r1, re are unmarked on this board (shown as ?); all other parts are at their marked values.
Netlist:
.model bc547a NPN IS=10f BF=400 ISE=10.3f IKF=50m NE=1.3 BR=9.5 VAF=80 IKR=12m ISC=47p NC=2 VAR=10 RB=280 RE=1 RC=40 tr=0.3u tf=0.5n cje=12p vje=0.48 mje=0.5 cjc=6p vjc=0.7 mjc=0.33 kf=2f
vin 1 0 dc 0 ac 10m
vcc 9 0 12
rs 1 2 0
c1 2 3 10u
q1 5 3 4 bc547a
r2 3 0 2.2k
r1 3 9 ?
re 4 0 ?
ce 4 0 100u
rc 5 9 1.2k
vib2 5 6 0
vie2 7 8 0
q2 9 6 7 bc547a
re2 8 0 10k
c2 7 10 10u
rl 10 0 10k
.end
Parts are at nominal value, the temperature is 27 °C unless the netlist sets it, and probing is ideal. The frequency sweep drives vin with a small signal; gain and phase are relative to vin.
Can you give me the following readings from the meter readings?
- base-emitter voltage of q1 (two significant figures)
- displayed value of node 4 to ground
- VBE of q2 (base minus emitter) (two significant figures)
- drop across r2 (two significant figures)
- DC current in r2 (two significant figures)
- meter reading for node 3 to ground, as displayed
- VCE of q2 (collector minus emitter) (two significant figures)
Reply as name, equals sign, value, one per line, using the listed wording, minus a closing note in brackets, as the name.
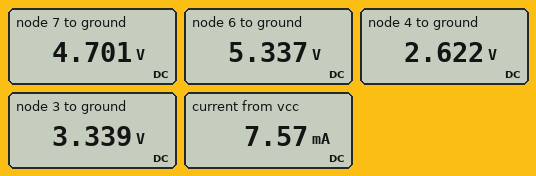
base-emitter voltage of q1 = 720 mV
displayed value of node 4 to ground = 2.622 V
VBE of q2 (base minus emitter) = 640 mV
drop across r2 = 3.3 V
DC current in r2 = 1.5 mA
meter reading for node 3 to ground, as displayed = 3.339 V
VCE of q2 (collector minus emitter) = 7.3 V
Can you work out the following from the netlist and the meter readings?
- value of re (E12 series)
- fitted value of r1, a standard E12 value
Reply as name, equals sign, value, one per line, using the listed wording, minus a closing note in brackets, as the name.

value of re = 470 Ω
fitted value of r1, a standard E12 value = 5.6 kΩ
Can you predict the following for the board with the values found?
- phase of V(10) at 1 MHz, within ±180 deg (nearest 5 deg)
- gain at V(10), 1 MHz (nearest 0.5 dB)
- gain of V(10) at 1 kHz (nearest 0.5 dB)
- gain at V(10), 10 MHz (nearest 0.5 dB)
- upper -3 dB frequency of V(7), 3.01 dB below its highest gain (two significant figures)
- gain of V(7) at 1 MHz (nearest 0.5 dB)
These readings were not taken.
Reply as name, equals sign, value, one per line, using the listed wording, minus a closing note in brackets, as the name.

phase of V(10) at 1 MHz, within ±180 deg = 130 deg
gain at V(10), 1 MHz = 39.0 dB
gain of V(10) at 1 kHz = 43.0 dB
gain at V(10), 10 MHz = 21.0 dB
upper -3 dB frequency of V(7), 3.01 dB below its highest gain = 800 kHz
gain of V(7) at 1 MHz = 39.0 dB
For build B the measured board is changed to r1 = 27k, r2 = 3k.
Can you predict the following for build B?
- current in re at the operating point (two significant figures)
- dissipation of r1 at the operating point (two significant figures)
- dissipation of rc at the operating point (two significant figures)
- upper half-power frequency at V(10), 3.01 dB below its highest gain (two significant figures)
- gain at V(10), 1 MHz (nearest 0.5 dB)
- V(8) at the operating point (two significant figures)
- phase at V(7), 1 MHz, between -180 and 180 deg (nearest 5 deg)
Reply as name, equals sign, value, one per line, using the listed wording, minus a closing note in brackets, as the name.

current in re at the operating point = 1.1 mA
dissipation of r1 at the operating point = 4.3 mW
dissipation of rc at the operating point = 1.5 mW
upper half-power frequency at V(10), 3.01 dB below its highest gain = 3.0 MHz
gain at V(10), 1 MHz = 32.5 dB
V(8) at the operating point = 10 V
phase at V(7), 1 MHz, between -180 and 180 deg = 160 deg
